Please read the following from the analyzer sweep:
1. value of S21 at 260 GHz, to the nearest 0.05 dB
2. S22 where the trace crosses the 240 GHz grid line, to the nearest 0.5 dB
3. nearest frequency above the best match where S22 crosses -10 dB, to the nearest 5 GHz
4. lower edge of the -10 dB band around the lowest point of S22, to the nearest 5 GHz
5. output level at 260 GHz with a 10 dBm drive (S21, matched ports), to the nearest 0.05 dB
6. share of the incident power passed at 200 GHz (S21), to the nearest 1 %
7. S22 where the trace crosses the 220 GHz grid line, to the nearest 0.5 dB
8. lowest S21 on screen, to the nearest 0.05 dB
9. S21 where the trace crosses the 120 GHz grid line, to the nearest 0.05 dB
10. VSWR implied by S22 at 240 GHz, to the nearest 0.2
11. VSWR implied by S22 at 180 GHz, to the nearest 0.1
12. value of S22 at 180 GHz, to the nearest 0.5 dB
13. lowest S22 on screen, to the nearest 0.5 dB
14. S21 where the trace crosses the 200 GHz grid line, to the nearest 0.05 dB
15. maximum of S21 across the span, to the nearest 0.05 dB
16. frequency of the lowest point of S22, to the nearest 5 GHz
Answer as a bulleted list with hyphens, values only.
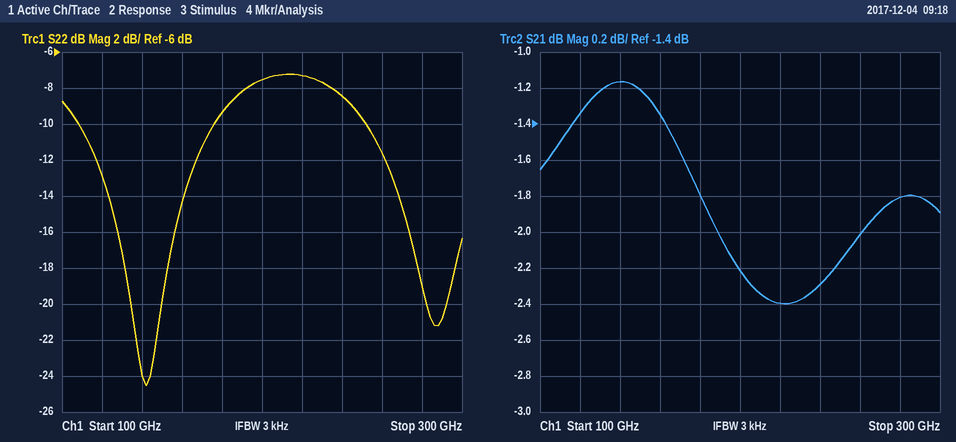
- -2.00 dB
- -8.5 dB
- 175 GHz
- 110 GHz
- 8.00 dBm
- 60 %
- -7.5 dB
- -2.40 dB
- -1.35 dB
- 2.2
- 2.0
- -9.5 dB
- -24.5 dB
- -2.20 dB
- -1.15 dB
- 140 GHz
